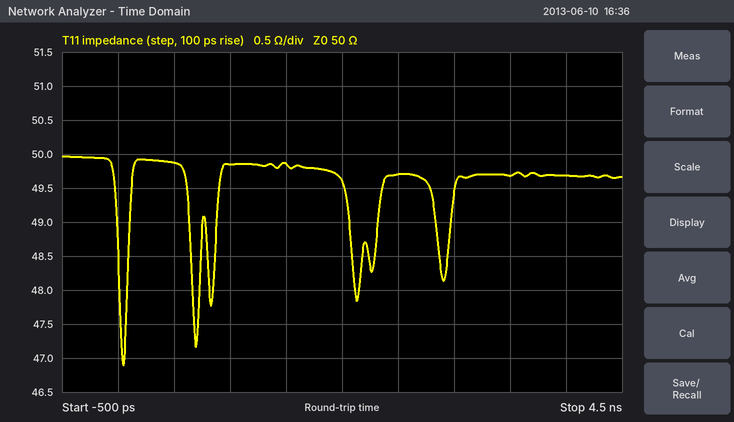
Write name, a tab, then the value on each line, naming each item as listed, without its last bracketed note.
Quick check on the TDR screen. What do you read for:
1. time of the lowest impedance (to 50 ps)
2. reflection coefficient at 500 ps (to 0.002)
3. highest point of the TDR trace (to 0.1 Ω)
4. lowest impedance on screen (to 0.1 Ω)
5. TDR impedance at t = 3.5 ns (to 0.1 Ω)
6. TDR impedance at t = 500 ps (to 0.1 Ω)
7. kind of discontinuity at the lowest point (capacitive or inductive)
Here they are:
time of the lowest impedance	50 ps
reflection coefficient at 500 ps	-0.002
highest point of the TDR trace	50.0 Ω
lowest impedance on screen	46.9 Ω
TDR impedance at t = 3.5 ns	49.7 Ω
TDR impedance at t = 500 ps	49.9 Ω
kind of discontinuity at the lowest point	capacitive
